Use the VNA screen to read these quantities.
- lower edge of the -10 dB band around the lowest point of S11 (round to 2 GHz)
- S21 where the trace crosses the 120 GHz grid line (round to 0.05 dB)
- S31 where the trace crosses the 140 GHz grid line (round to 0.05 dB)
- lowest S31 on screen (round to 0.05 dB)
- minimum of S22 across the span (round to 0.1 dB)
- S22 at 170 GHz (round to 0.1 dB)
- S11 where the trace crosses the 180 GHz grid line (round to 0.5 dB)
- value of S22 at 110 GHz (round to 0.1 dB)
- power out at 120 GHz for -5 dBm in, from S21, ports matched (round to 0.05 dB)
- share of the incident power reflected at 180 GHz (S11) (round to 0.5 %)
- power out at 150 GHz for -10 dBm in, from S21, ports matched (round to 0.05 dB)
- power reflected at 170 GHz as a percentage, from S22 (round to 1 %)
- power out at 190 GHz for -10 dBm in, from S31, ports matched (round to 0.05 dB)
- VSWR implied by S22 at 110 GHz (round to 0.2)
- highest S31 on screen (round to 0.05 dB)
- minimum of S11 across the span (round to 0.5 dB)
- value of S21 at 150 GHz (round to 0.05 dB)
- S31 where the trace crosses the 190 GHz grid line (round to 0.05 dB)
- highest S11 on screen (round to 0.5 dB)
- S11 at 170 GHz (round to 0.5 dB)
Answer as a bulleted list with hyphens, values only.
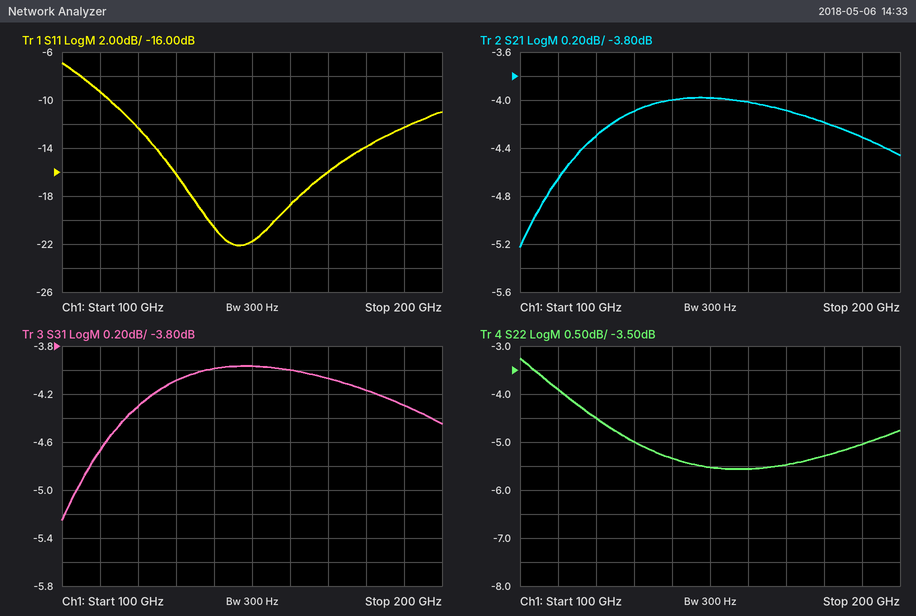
- 112 GHz
- -4.30 dB
- -4.00 dB
- -5.25 dB
- -5.6 dB
- -5.5 dB
- -14.0 dB
- -3.9 dB
- -9.30 dBm
- 4.0 %
- -14.00 dBm
- 28 %
- -14.30 dBm
- 4.6
- -3.95 dB
- -22.0 dB
- -4.00 dB
- -4.30 dB
- -7.0 dB
- -16.0 dB
